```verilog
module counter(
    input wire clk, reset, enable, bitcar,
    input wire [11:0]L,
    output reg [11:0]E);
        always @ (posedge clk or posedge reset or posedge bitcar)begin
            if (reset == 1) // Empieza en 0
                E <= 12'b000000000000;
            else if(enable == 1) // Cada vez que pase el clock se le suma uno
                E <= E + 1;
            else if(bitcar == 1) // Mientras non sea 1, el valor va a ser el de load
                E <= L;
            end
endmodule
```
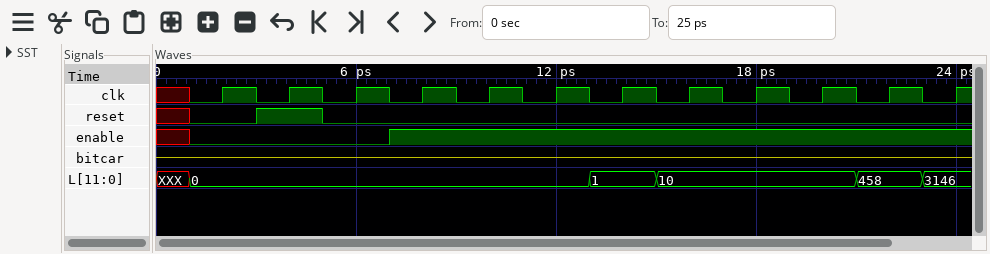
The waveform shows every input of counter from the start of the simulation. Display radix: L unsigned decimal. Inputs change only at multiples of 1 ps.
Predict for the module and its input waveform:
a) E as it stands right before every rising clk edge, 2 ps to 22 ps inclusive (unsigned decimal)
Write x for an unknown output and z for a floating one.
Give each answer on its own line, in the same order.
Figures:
x, 0, 0, 0, 1, 2, 3, 4, 5, 6, 7
